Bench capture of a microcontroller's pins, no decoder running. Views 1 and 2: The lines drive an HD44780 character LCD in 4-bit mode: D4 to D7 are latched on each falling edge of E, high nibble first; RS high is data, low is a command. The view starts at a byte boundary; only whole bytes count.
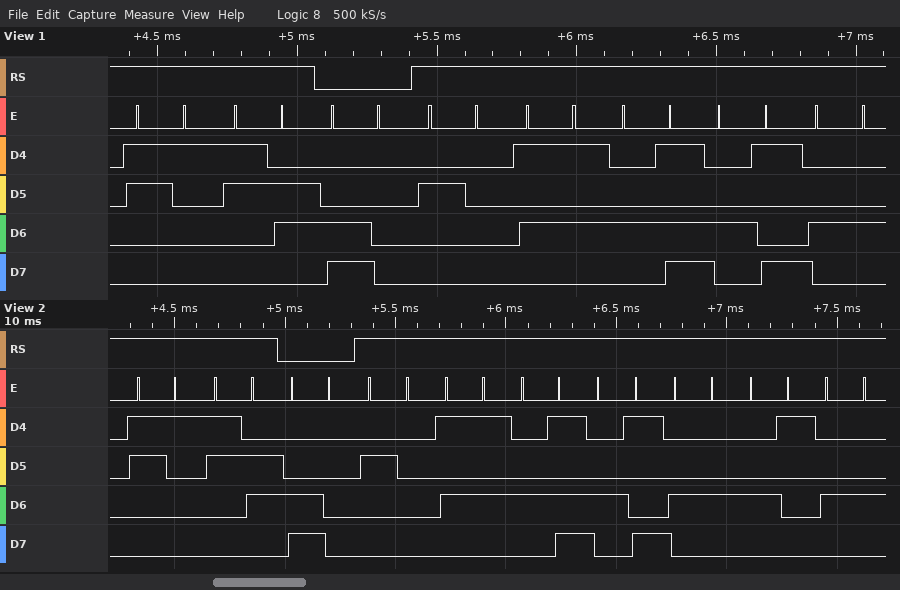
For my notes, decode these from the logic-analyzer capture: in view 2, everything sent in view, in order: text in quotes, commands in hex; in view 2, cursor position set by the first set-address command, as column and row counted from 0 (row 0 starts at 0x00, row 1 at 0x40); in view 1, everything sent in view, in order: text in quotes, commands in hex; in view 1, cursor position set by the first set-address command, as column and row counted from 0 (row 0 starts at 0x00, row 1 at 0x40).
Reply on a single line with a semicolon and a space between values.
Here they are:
"16" 0xC0 " UMIDAD"; column 0, row 1; "16" 0xC0 " UMID"; column 0, row 1
